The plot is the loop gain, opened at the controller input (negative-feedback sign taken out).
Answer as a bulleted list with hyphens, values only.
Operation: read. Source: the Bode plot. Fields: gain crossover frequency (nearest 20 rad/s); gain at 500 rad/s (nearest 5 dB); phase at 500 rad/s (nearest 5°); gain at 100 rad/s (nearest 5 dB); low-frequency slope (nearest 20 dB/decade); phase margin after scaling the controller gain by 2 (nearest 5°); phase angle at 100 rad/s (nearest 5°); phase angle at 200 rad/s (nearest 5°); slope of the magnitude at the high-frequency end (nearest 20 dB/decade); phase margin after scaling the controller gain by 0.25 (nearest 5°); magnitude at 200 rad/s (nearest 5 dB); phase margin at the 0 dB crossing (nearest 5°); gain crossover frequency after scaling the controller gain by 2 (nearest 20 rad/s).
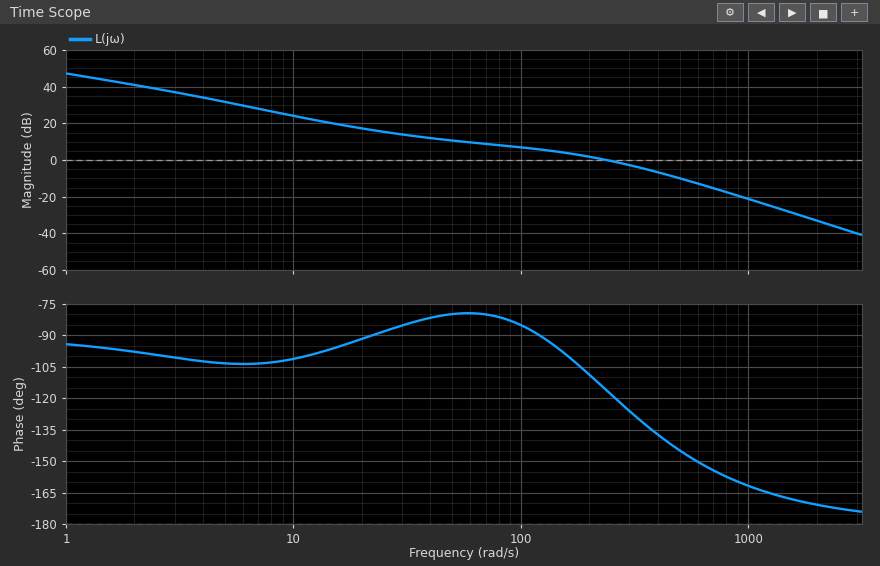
- 240 rad/s
- -10 dB
- -145°
- 5 dB
- -20 dB/decade
- 45°
- -85°
- -110°
- -40 dB/decade
- 100°
- 0 dB
- 65°
- 380 rad/s
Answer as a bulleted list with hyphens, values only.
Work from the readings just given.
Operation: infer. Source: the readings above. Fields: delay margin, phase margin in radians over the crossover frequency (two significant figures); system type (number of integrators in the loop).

- 0.0047 s
- 1
